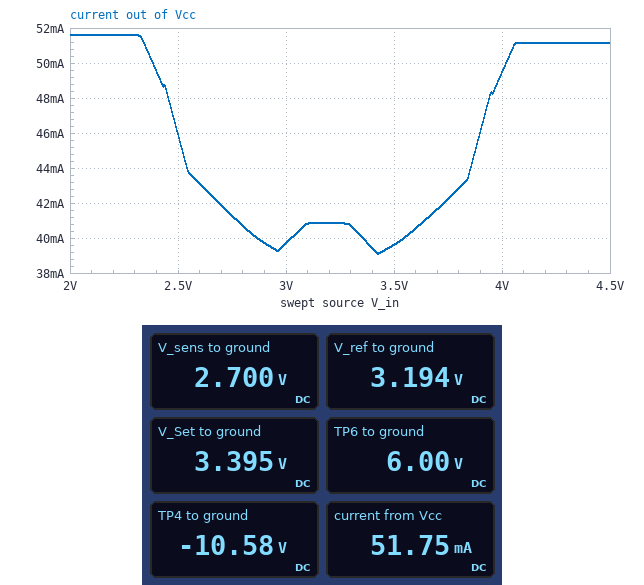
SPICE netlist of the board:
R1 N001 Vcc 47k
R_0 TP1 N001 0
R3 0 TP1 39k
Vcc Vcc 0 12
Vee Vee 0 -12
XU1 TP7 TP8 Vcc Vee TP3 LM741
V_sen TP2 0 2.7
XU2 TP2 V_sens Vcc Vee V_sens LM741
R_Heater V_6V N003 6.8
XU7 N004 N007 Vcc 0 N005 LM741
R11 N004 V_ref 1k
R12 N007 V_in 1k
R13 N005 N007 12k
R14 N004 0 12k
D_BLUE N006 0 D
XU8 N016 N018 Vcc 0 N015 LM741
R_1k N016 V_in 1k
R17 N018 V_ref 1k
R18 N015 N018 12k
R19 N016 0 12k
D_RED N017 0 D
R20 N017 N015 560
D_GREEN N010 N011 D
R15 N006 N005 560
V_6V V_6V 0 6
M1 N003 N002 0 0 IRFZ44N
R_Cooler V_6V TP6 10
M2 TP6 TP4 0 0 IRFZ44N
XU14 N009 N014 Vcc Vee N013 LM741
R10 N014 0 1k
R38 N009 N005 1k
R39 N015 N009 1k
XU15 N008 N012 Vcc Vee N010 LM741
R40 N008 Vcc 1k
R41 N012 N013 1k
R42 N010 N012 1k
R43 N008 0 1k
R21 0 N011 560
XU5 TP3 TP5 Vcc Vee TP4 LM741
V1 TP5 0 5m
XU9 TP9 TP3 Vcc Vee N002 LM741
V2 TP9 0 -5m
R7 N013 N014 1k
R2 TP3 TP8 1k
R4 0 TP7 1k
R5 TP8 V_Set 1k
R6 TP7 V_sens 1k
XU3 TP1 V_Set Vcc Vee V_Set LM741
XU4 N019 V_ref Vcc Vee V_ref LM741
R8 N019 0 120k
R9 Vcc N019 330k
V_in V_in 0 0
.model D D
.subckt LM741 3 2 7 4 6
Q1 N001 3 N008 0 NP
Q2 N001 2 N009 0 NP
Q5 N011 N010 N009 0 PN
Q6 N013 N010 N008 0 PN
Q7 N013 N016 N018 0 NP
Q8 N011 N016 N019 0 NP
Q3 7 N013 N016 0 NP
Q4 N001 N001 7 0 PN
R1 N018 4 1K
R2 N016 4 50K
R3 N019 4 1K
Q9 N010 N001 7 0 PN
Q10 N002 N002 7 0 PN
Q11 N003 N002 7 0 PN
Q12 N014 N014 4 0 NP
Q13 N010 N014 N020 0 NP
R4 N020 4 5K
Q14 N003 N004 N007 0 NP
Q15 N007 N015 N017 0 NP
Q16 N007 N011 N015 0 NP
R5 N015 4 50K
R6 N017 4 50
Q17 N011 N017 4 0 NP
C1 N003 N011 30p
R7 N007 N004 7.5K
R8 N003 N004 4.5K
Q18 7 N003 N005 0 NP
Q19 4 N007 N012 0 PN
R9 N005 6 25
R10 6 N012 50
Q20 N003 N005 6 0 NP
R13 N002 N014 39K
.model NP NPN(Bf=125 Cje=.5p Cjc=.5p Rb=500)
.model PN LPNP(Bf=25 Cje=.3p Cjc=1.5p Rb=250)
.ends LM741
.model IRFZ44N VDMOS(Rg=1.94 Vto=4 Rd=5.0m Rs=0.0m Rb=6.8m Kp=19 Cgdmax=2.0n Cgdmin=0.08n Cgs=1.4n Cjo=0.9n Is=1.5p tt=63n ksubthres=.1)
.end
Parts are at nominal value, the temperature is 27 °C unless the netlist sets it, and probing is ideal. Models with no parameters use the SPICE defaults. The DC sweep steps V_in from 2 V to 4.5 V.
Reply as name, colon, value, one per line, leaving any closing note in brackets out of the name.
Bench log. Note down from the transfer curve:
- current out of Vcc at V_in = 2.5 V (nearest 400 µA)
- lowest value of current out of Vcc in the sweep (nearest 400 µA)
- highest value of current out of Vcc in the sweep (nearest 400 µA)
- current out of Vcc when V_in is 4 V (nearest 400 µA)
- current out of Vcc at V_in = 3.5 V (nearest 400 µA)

current out of Vcc at V_in = 2.5 V: 46.0 mA
lowest value of current out of Vcc in the sweep: 39.2 mA
highest value of current out of Vcc in the sweep: 51.6 mA
current out of Vcc when V_in is 4 V: 49.6 mA
current out of Vcc at V_in = 3.5 V: 39.6 mA
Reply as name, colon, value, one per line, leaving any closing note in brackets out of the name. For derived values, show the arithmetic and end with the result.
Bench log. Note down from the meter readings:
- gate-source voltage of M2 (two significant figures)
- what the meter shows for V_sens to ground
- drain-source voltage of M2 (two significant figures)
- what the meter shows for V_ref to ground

gate-source voltage of M2: -10.58 V = -11 V
what the meter shows for V_sens to ground: 2.700 V
drain-source voltage of M2: 6 V = 6.0 V
what the meter shows for V_ref to ground: 3.194 V
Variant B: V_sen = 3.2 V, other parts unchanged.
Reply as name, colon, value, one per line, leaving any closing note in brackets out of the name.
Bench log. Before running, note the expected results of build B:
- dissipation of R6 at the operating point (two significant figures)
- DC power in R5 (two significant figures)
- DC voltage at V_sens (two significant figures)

dissipation of R6 at the operating point: 2.6 mW
DC power in R5: 3.2 mW
DC voltage at V_sens: 3.2 V
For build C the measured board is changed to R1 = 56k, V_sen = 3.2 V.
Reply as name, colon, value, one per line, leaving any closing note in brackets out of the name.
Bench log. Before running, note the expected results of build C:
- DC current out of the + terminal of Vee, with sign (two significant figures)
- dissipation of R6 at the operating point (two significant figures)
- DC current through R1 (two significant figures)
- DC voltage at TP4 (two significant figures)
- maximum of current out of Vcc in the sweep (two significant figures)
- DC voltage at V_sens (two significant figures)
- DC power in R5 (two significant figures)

DC current out of the + terminal of Vee, with sign: -13 mA
dissipation of R6 at the operating point: 2.6 mW
DC current through R1: 160 µA
DC voltage at TP4: 12 V
maximum of current out of Vcc in the sweep: 51 mA
DC voltage at V_sens: 3.2 V
DC power in R5: 1.6 mW
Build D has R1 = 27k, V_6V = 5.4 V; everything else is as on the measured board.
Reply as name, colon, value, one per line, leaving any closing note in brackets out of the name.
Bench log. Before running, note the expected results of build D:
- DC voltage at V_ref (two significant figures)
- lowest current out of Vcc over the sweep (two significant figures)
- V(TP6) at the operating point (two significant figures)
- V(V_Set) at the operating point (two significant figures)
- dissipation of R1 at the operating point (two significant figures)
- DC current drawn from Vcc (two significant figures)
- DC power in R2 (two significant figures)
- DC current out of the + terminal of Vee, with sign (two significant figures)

DC voltage at V_ref: 3.2 V
lowest current out of Vcc over the sweep: 42 mA
V(TP6) at the operating point: 5.4 V
V(V_Set) at the operating point: 5.9 V
dissipation of R1 at the operating point: 1.4 mW
DC current drawn from Vcc: 54 mA
DC power in R2: 21 mW
DC current out of the + terminal of Vee, with sign: -17 mA
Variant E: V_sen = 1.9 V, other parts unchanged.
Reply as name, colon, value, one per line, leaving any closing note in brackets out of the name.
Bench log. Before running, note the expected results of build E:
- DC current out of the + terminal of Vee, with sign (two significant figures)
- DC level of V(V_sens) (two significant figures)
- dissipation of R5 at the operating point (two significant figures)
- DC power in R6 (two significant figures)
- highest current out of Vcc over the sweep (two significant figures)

DC current out of the + terminal of Vee, with sign: -15 mA
DC level of V(V_sens): 1.9 V
dissipation of R5 at the operating point: 6.0 mW
DC power in R6: 900 µW
highest current out of Vcc over the sweep: 52 mA
